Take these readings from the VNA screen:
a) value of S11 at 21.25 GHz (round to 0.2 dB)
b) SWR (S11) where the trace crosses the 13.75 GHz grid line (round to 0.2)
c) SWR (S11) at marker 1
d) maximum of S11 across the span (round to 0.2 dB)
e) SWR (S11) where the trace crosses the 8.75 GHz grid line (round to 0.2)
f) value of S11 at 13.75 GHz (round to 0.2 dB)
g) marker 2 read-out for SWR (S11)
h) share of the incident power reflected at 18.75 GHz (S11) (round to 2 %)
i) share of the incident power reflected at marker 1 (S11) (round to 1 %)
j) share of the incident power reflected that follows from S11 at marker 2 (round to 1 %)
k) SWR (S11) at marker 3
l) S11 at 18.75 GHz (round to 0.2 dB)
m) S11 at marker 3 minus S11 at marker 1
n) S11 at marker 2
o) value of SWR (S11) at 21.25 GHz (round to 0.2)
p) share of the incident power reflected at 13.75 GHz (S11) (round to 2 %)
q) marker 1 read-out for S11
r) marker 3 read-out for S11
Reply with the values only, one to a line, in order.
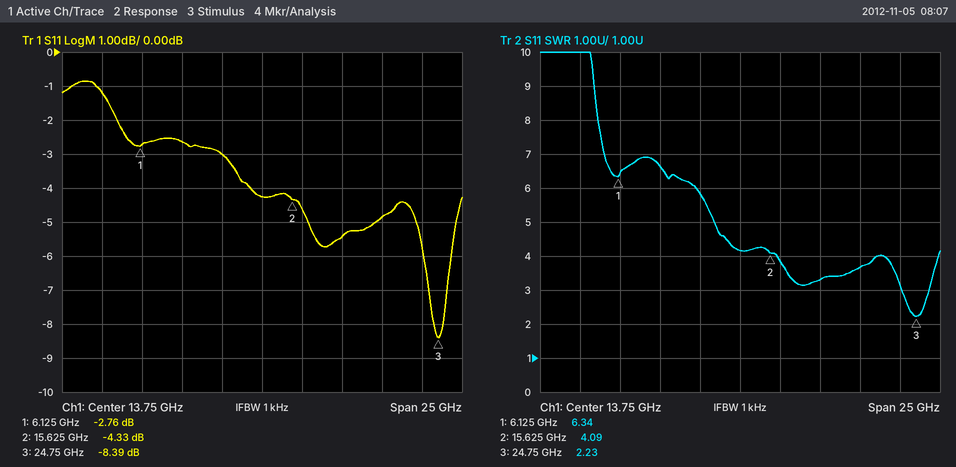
-4.8 dB
4.2
6.34
-0.8 dB
6.6
-4.2 dB
4.09
28 %
53 %
37 %
2.23
-5.4 dB
-5.63 dB
-4.33 dB
3.6
38 %
-2.76 dB
-8.39 dB
